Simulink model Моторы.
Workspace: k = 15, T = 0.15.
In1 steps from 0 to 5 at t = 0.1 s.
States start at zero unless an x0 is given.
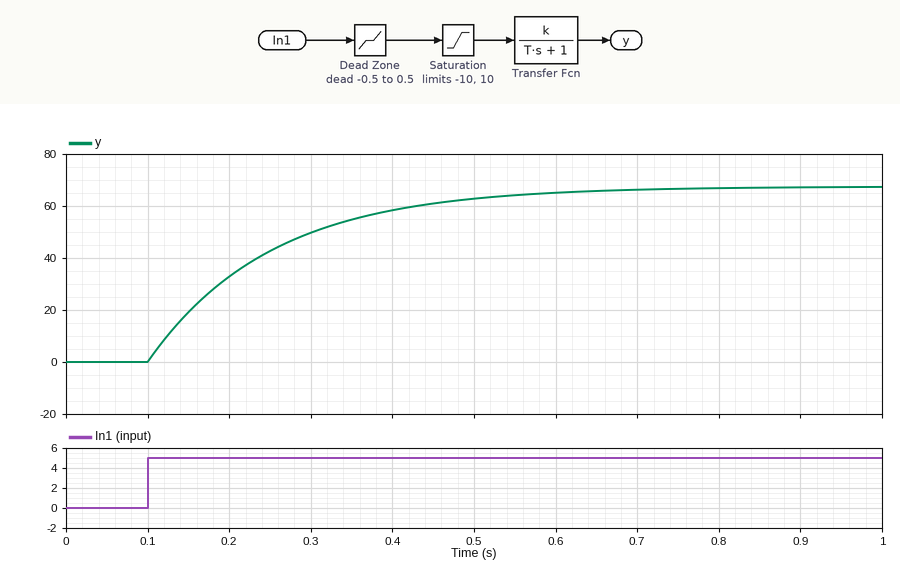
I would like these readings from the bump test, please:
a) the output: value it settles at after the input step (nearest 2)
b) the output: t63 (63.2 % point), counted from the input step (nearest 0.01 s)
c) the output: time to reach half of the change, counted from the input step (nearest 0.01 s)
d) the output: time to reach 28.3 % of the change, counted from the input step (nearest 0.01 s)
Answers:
68
0.15 s
0.10 s
0.05 s
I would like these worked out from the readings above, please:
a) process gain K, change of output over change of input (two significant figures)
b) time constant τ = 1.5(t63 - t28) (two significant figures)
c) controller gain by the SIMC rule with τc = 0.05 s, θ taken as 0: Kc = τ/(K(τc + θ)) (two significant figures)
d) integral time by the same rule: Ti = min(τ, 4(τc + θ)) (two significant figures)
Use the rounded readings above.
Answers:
14
0.15 s
0.21
0.15 s
